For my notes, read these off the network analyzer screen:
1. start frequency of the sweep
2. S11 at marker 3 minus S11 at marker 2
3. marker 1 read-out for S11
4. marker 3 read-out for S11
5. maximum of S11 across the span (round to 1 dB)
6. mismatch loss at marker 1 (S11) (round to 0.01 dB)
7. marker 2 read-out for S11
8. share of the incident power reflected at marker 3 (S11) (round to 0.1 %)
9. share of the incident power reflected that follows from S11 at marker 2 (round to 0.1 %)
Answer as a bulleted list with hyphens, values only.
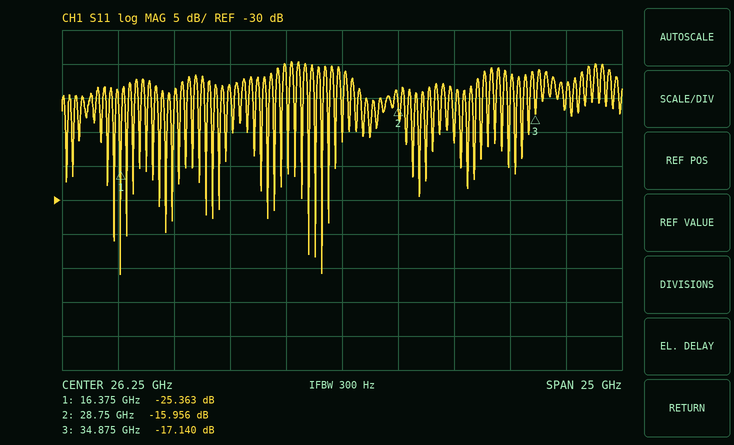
- 13.75 GHz
- -1.184 dB
- -25.363 dB
- -17.140 dB
- -10 dB
- 0.01 dB
- -15.956 dB
- 1.9 %
- 2.5 %
